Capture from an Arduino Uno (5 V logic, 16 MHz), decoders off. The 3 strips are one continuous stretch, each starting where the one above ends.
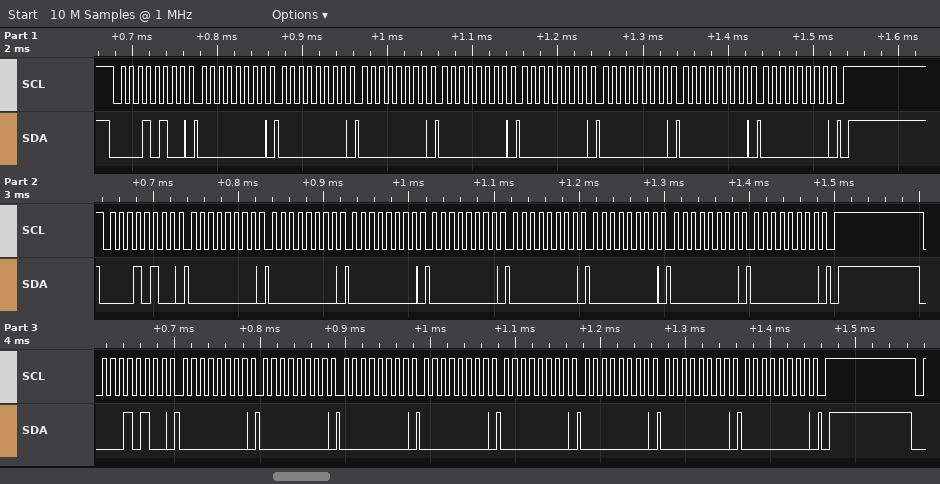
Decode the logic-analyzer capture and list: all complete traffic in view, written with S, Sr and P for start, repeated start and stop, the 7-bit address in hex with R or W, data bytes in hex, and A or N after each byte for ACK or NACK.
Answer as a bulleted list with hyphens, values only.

- S 0AW A 00 A 00 A 00 A 00 A 00 A 00 A 00 A 00 A P S 0AW A 00 A 00 A 00 A 00 A 00 A 00 A 00 A 00 A P S 0AW A 00 A 00 A 00 A 00 A 00 A 00 A 00 A 00 A P
